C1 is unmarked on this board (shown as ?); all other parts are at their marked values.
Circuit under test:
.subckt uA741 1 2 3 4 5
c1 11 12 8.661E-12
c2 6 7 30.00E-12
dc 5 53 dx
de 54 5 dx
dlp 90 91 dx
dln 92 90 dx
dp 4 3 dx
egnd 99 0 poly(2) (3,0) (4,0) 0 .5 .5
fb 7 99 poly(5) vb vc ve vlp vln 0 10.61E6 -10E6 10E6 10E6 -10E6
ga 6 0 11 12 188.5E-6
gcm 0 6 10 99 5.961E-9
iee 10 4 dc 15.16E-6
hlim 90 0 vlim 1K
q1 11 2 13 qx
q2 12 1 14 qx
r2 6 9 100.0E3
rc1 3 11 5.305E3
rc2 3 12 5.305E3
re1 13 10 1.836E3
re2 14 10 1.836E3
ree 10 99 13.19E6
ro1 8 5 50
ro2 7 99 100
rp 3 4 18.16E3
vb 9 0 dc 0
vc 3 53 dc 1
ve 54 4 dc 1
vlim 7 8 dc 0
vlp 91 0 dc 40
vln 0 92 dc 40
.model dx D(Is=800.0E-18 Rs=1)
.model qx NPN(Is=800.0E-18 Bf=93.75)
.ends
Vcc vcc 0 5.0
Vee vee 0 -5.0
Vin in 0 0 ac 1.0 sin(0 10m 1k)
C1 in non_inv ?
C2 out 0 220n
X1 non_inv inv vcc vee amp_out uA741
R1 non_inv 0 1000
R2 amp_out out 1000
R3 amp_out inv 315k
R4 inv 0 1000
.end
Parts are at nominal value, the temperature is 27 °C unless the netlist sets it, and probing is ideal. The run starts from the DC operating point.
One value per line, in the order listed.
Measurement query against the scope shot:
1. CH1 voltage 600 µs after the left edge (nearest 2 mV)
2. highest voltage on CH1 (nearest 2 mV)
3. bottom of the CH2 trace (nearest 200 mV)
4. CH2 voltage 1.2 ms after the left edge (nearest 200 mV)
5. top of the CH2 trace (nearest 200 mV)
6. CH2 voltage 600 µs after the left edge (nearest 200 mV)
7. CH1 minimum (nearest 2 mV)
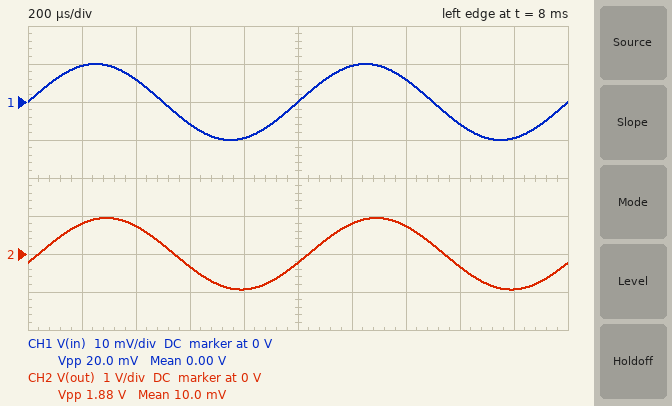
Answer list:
-6 mV
10 mV
-1.0 V
800 mV
1.0 V
-400 mV
-10 mV
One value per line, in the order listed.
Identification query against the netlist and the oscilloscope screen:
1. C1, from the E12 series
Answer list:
100 nF
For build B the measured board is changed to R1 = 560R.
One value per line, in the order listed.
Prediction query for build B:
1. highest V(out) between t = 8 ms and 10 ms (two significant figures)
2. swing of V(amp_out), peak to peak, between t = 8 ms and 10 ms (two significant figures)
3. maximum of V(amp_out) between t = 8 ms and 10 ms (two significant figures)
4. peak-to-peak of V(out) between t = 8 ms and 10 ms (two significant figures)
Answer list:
600 mV
2.0 V
1.0 V
1.2 V
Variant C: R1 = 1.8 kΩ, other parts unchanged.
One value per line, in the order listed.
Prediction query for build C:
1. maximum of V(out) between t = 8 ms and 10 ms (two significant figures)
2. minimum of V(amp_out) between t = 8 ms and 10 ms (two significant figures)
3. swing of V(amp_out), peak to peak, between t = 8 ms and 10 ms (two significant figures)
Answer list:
1.3 V
-2.3 V
4.5 V
